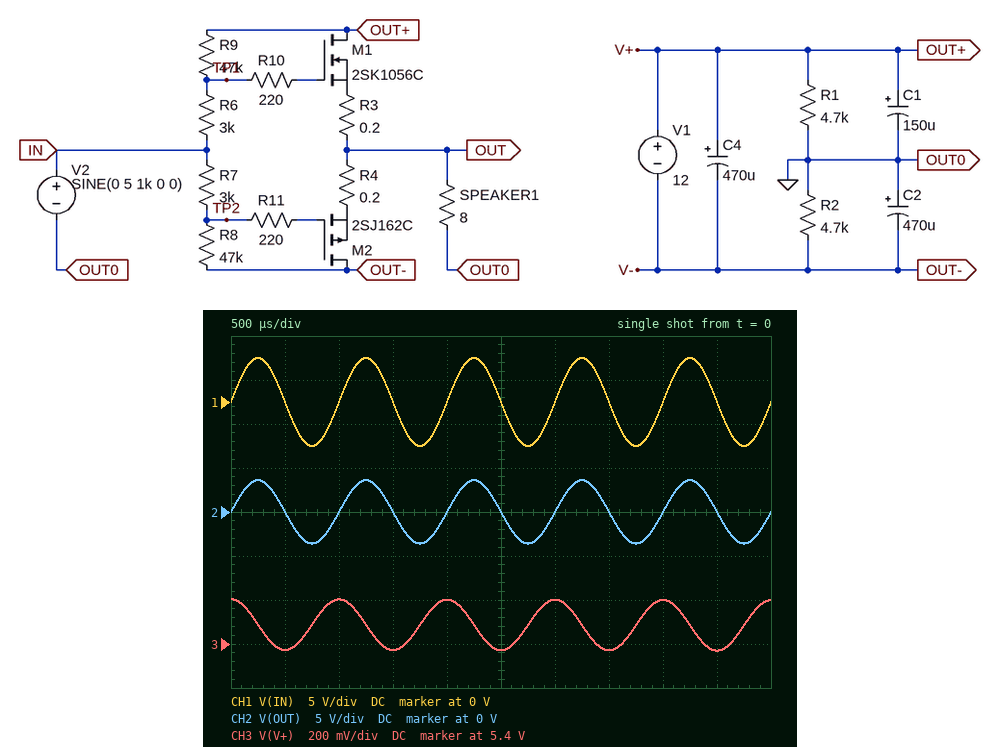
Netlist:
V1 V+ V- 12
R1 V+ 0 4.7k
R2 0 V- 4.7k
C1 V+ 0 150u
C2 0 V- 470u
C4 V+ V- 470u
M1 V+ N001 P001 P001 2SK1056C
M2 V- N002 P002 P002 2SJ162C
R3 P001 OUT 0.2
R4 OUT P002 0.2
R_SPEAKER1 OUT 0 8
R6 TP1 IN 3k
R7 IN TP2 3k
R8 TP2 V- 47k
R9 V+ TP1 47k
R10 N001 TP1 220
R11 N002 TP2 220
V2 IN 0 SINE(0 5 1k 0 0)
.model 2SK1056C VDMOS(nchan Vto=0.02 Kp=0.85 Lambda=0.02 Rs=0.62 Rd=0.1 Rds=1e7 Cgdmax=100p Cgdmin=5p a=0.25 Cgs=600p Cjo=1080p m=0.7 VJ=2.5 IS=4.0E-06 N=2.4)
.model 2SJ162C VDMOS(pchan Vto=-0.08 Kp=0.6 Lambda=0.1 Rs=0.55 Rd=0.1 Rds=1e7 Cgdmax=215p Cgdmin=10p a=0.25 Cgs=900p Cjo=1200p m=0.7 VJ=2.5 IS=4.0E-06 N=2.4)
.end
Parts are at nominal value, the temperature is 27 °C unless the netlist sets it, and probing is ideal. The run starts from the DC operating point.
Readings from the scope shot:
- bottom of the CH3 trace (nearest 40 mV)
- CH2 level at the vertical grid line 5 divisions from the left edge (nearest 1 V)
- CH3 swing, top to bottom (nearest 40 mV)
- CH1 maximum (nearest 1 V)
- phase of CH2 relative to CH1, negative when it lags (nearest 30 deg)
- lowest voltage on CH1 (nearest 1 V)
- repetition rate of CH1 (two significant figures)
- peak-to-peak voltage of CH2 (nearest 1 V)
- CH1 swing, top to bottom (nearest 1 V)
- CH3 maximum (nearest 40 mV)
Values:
5.36 V
0 V
240 mV
5 V
0 deg
-5 V
1.0 kHz
7 V
10 V
5.60 V
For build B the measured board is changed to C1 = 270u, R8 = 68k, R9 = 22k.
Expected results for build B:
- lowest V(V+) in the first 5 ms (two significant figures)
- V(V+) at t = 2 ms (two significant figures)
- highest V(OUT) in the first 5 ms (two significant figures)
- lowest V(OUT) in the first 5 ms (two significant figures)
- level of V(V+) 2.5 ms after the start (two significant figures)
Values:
3.0 V
3.2 V
2.7 V
-3.7 V
3.1 V
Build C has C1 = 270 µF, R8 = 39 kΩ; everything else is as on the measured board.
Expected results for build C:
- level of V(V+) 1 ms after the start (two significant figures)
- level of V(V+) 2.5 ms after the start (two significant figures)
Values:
6.1 V
5.9 V
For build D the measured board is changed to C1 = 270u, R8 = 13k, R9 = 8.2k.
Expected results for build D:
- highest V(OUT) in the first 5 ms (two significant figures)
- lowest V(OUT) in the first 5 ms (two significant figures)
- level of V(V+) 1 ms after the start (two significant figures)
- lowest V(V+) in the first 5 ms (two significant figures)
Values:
3.4 V
-3.4 V
5.0 V
4.8 V
